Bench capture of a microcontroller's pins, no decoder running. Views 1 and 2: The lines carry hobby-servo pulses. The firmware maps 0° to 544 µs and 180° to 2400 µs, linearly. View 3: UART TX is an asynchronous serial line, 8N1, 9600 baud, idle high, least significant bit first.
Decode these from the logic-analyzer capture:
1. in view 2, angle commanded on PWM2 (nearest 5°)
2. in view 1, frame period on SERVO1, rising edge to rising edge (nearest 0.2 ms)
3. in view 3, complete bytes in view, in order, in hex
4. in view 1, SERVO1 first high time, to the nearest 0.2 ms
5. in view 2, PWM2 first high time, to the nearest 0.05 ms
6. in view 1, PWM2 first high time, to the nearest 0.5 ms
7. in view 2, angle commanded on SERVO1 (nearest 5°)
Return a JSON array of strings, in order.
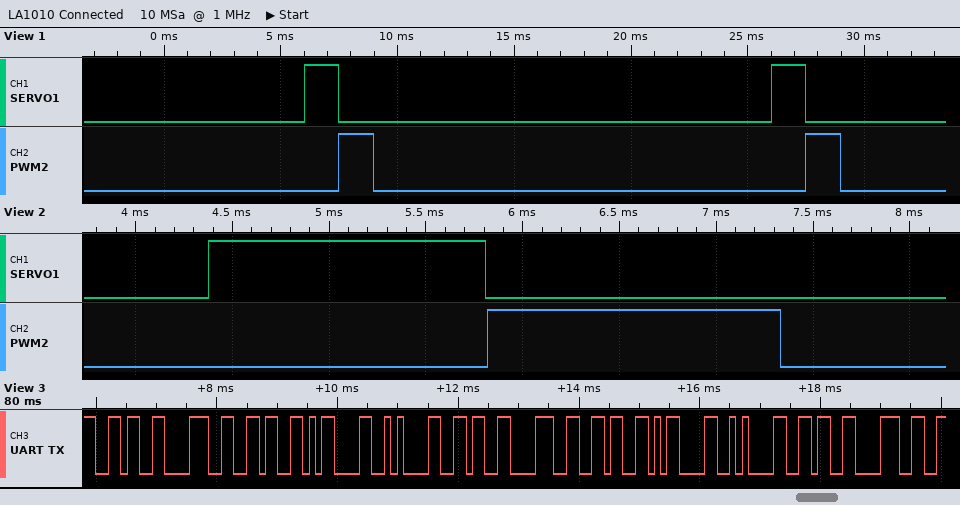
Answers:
["95°", "20.0 ms", "36 38 36 0D 0A 36 38 36 0D 0A 36 38", "1.4 ms", "1.50 ms", "1.5 ms", "85°"]
